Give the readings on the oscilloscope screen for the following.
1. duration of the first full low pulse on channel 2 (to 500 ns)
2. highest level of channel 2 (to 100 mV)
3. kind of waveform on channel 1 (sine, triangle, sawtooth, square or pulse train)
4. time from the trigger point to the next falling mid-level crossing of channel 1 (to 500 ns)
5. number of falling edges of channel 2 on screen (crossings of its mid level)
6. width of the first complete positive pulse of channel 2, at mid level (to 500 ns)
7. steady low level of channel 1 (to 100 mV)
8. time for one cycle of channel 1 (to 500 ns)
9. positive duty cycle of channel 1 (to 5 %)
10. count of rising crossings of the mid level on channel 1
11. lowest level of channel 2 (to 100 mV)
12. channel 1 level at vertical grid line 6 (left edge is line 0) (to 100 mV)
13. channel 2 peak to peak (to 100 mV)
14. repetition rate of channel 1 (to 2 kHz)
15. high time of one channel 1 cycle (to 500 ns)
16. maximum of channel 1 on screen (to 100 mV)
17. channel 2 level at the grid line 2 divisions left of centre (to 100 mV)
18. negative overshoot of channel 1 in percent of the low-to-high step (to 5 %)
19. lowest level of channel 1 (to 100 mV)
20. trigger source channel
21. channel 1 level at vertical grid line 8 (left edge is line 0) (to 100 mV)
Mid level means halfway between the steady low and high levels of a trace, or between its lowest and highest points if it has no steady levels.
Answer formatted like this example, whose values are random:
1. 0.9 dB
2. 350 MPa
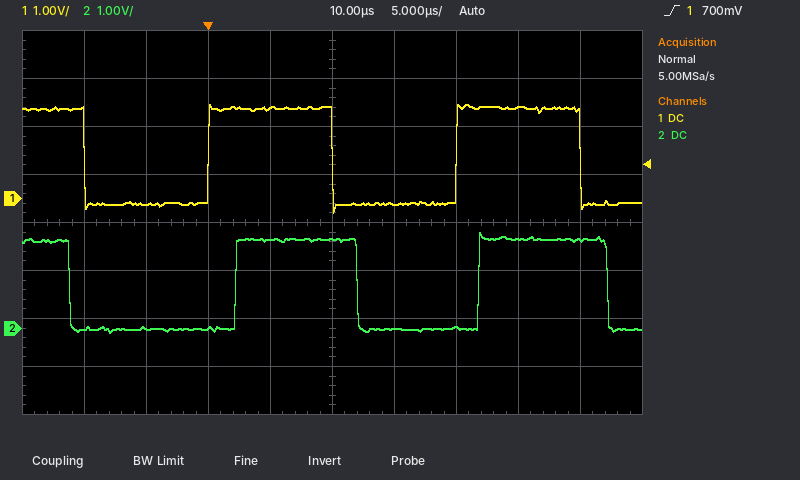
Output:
1. 13.5 µs
2. 2.0 V
3. square
4. 10.0 µs
5. 3
6. 10.0 µs
7. -100 mV
8. 20.0 µs
9. 50 %
10. 2
11. -100 mV
12. -100 mV
13. 2.1 V
14. 50 kHz
15. 10.0 µs
16. 2.0 V
17. 0.0 V
18. 10 %
19. -300 mV
20. channel 1
21. 1.9 V
